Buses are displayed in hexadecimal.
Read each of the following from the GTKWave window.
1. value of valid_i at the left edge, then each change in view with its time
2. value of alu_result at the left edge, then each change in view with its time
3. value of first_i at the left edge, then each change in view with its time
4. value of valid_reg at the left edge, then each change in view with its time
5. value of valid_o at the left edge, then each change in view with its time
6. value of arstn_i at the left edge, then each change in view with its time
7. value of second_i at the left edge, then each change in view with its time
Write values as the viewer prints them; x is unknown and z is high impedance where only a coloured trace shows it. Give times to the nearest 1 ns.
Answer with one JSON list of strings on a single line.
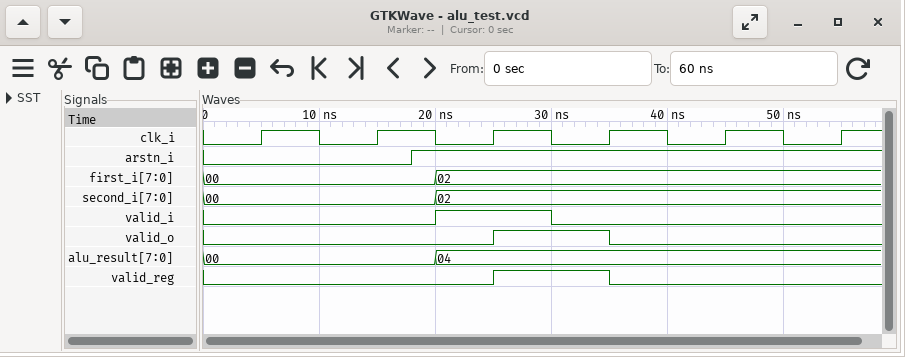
["0, 1 at 20 ns, 0 at 30 ns", "00, 04 at 20 ns", "00, 02 at 20 ns", "0, 1 at 25 ns, 0 at 35 ns", "0, 1 at 25 ns, 0 at 35 ns", "0, 1 at 18 ns", "00, 02 at 20 ns"]
